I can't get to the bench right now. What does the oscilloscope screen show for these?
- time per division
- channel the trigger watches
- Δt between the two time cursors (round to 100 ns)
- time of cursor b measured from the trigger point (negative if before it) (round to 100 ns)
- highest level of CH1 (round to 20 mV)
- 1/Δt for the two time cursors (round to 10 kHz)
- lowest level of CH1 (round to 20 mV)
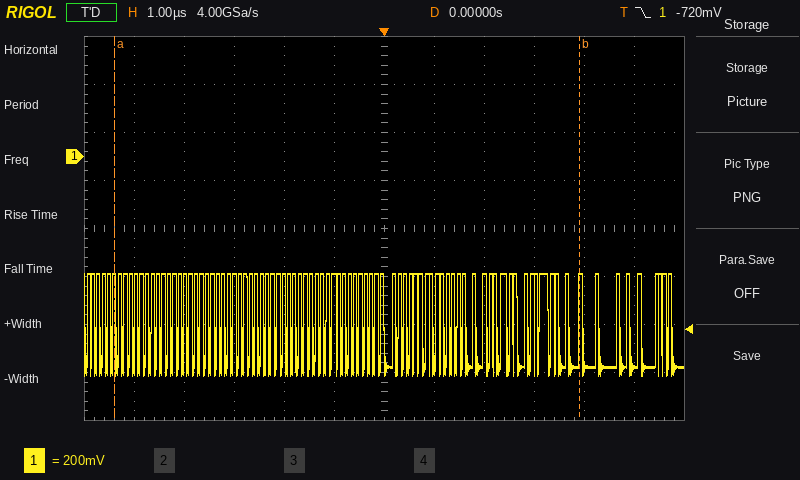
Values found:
1 µs
CH1
9.3 µs
+3.9 µs
-480 mV
110 kHz
-920 mV
